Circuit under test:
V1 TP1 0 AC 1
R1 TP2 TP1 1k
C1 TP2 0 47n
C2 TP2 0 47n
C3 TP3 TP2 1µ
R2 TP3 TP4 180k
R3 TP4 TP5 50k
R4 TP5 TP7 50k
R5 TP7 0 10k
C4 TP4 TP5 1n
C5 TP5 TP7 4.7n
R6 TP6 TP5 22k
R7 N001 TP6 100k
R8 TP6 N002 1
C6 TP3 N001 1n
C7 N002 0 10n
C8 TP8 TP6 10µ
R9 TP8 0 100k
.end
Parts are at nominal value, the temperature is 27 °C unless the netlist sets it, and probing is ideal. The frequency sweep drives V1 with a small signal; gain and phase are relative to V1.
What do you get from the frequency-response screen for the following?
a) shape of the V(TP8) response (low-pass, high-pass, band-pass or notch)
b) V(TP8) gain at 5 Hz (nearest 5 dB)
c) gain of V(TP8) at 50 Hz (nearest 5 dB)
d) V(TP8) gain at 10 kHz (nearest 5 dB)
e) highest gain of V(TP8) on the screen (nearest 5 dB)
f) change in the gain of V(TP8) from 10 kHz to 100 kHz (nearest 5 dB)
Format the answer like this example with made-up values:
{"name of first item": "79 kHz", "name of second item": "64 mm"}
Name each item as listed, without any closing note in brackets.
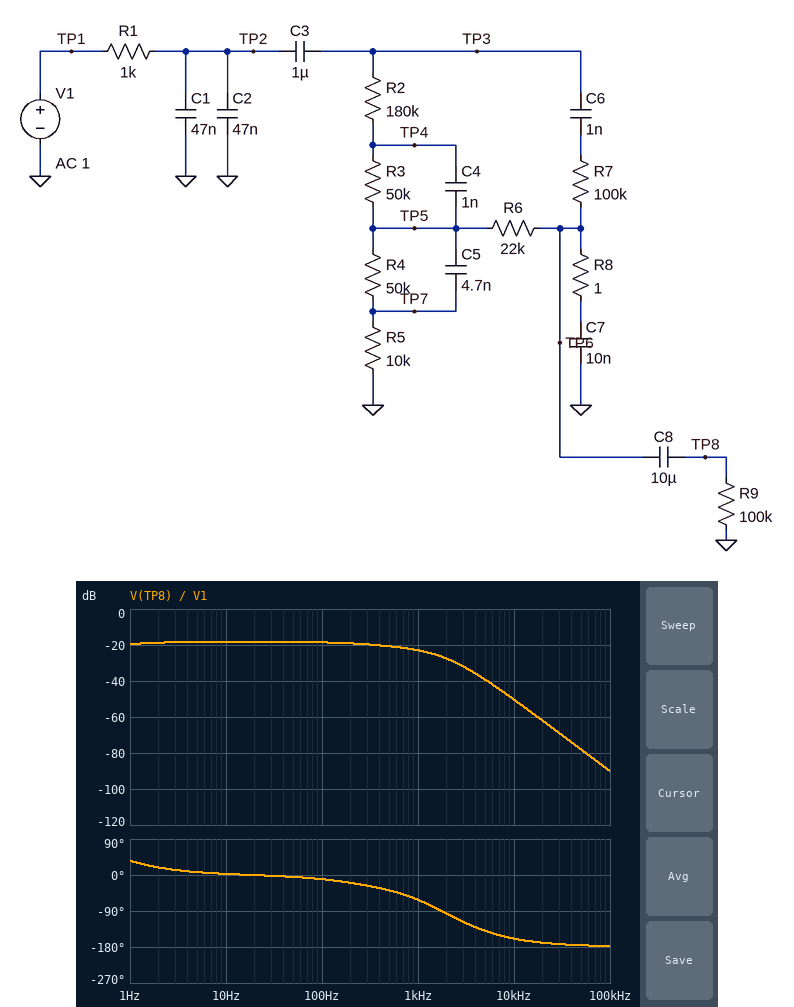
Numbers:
{"shape of the V(TP8) response": "low-pass", "V(TP8) gain at 5 Hz": "-20 dB", "gain of V(TP8) at 50 Hz": "-20 dB", "V(TP8) gain at 10 kHz": "-50 dB", "highest gain of V(TP8) on the screen": "-20 dB", "change in the gain of V(TP8) from 10 kHz to 100 kHz": "-40 dB"}
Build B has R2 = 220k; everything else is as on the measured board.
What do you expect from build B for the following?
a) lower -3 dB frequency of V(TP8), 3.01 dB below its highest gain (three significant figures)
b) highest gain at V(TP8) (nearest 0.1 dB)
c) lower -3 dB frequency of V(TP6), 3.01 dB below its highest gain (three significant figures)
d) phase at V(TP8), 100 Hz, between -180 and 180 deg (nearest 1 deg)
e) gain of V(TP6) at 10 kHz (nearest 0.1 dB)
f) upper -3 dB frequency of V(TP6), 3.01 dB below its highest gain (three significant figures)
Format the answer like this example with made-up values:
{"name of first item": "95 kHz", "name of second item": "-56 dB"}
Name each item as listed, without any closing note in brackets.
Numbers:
{"lower -3 dB frequency of V(TP8), 3.01 dB below its highest gain": "530 mHz", "highest gain at V(TP8)": "-19.5 dB", "lower -3 dB frequency of V(TP6), 3.01 dB below its highest gain": "482 mHz", "phase at V(TP8), 100 Hz, between -180 and 180 deg": "-9 deg", "gain of V(TP6) at 10 kHz": "-50.6 dB", "upper -3 dB frequency of V(TP6), 3.01 dB below its highest gain": "816 Hz"}
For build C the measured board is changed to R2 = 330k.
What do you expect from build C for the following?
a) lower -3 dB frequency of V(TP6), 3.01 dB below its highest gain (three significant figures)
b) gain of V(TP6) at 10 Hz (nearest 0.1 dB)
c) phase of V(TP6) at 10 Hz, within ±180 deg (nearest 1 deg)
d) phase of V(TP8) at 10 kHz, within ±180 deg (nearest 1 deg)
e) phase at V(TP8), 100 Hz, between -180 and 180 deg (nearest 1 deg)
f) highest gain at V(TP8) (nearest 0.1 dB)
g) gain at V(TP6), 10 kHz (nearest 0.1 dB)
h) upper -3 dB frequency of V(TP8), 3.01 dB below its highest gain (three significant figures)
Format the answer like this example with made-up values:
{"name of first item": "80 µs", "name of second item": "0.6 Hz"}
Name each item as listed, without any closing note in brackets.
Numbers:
{"lower -3 dB frequency of V(TP6), 3.01 dB below its highest gain": "346 mHz", "gain of V(TP6) at 10 Hz": "-22.1 dB", "phase of V(TP6) at 10 Hz, within ±180 deg": "1 deg", "phase of V(TP8) at 10 kHz, within ±180 deg": "-158 deg", "phase at V(TP8), 100 Hz, between -180 and 180 deg": "-5 deg", "highest gain at V(TP8)": "-22.0 dB", "gain at V(TP6), 10 kHz": "-50.9 dB", "upper -3 dB frequency of V(TP8), 3.01 dB below its highest gain": "1.28 kHz"}
